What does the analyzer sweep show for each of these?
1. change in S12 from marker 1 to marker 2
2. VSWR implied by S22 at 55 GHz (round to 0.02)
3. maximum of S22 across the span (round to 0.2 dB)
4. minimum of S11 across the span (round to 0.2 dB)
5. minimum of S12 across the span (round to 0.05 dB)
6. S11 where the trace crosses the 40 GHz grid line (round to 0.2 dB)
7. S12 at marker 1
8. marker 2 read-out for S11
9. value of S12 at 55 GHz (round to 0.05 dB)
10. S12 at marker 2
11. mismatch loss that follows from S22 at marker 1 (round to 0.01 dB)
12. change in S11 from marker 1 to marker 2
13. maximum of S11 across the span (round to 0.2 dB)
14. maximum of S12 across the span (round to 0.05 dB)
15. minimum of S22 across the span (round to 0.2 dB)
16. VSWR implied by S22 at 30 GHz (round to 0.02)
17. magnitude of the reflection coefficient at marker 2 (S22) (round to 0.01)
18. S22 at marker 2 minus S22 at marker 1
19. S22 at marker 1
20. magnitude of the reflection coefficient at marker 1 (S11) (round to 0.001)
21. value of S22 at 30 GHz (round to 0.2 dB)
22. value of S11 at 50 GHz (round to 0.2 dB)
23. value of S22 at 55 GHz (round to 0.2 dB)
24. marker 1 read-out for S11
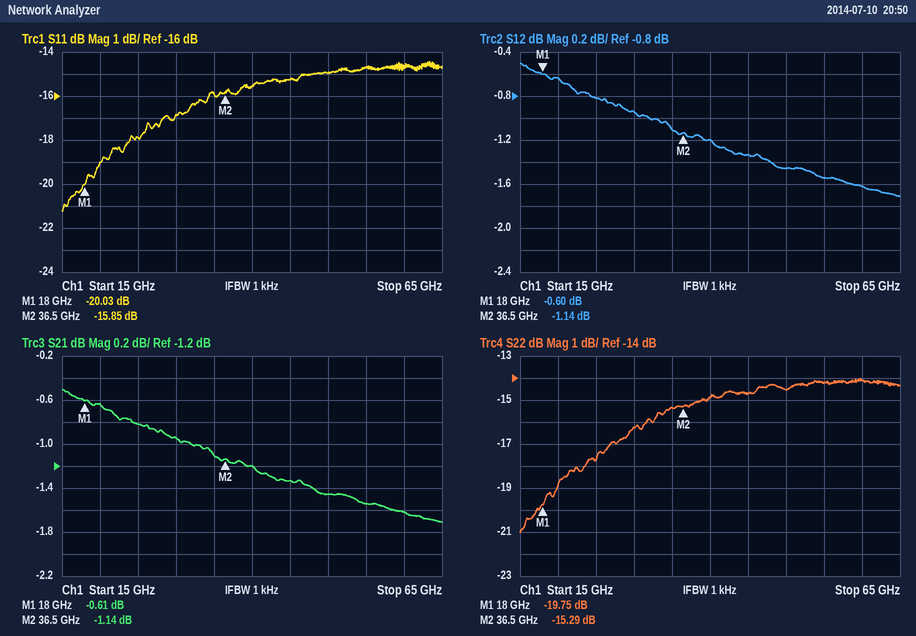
-0.54 dB
1.48
-14.0 dB
-21.2 dB
-1.70 dB
-15.6 dB
-0.60 dB
-15.85 dB
-1.55 dB
-1.14 dB
0.05 dB
4.18 dB
-14.4 dB
-0.50 dB
-21.0 dB
1.36
0.17
4.46 dB
-19.75 dB
0.100
-16.2 dB
-15.0 dB
-14.2 dB
-20.03 dB
